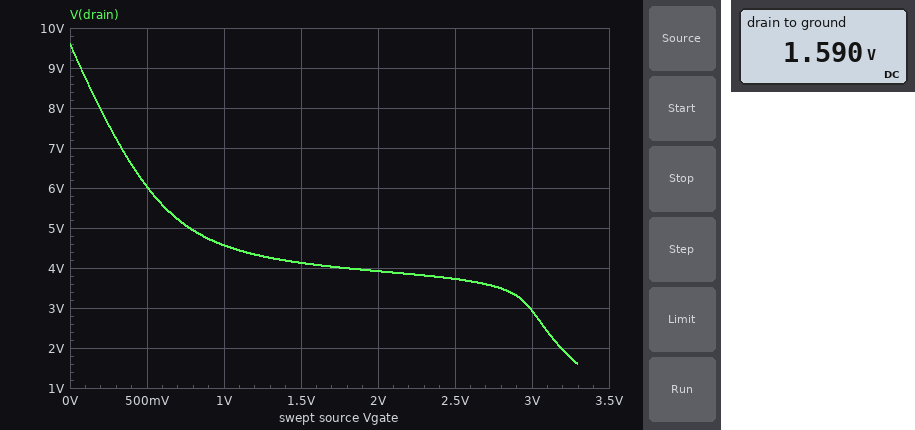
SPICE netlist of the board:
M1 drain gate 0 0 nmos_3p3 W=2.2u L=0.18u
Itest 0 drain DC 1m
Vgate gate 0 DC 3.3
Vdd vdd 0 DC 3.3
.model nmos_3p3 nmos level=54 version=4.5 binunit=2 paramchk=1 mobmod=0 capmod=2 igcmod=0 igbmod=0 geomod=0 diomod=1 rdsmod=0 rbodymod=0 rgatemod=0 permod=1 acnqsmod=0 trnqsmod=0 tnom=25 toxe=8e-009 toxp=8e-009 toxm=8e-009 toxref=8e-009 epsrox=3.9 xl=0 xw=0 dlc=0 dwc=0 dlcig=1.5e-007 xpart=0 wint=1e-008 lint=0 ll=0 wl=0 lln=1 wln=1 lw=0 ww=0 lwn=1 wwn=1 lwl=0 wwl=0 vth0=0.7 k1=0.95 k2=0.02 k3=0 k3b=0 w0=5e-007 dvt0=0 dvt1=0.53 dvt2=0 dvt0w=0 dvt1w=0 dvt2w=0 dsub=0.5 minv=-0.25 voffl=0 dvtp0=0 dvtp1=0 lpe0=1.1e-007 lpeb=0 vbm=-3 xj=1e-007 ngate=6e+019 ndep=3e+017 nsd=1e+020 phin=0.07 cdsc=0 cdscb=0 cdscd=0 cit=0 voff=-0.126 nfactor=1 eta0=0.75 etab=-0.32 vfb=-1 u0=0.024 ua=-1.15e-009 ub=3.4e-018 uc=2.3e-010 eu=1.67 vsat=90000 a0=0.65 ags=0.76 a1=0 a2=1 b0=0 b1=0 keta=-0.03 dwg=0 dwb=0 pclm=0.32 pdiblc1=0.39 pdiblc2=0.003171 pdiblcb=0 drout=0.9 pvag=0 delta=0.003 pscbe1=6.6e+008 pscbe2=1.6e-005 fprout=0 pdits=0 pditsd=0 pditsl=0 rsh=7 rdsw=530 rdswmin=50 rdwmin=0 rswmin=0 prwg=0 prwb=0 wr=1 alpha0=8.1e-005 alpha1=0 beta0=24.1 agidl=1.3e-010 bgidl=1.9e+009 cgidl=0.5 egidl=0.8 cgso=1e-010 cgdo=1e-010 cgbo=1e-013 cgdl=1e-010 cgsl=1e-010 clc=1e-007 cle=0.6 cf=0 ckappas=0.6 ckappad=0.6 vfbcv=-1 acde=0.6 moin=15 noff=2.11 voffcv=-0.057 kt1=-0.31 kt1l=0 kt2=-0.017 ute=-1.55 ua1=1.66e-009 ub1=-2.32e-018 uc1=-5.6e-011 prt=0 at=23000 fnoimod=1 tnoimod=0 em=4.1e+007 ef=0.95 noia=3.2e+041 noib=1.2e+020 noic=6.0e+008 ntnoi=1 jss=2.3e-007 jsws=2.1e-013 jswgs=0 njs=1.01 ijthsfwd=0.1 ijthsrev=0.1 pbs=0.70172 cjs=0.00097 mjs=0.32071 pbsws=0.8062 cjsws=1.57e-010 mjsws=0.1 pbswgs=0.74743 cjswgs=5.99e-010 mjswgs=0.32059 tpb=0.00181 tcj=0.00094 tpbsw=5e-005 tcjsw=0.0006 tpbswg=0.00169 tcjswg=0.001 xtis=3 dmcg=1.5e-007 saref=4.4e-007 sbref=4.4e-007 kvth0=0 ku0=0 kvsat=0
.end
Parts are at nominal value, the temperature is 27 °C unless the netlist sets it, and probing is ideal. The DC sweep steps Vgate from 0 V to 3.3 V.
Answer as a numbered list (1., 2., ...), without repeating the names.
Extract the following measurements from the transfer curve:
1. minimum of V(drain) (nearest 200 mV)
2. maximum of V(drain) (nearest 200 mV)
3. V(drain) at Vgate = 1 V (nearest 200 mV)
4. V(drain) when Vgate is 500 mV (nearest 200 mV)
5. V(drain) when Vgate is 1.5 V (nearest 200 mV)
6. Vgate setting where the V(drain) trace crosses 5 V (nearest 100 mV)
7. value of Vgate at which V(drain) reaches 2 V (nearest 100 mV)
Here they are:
1. 1.6 V
2. 9.6 V
3. 4.6 V
4. 6.0 V
5. 4.2 V
6. 800 mV
7. 3.2 V
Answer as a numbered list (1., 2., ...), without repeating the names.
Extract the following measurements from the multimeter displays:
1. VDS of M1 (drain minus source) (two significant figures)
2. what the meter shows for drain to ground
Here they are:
1. 1.6 V
2. 1.590 V
